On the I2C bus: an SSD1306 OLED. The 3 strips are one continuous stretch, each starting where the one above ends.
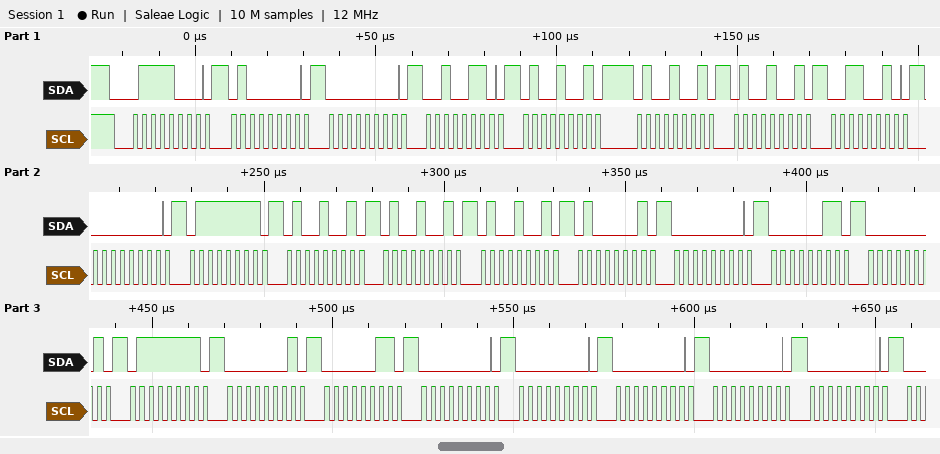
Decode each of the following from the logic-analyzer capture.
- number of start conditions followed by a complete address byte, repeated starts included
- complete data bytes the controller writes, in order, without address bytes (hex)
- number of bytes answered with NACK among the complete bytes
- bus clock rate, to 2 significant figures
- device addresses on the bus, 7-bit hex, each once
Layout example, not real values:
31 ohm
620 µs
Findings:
1
40 00 26 49 49 49 32 00 7F 49 49 49 41 00 03 01 7F 01 03 00 00 00 00 00
0
400 kHz
0x3C
